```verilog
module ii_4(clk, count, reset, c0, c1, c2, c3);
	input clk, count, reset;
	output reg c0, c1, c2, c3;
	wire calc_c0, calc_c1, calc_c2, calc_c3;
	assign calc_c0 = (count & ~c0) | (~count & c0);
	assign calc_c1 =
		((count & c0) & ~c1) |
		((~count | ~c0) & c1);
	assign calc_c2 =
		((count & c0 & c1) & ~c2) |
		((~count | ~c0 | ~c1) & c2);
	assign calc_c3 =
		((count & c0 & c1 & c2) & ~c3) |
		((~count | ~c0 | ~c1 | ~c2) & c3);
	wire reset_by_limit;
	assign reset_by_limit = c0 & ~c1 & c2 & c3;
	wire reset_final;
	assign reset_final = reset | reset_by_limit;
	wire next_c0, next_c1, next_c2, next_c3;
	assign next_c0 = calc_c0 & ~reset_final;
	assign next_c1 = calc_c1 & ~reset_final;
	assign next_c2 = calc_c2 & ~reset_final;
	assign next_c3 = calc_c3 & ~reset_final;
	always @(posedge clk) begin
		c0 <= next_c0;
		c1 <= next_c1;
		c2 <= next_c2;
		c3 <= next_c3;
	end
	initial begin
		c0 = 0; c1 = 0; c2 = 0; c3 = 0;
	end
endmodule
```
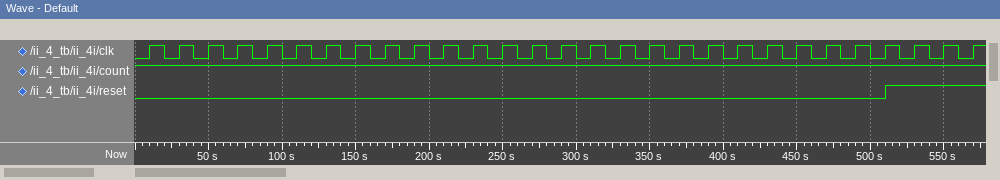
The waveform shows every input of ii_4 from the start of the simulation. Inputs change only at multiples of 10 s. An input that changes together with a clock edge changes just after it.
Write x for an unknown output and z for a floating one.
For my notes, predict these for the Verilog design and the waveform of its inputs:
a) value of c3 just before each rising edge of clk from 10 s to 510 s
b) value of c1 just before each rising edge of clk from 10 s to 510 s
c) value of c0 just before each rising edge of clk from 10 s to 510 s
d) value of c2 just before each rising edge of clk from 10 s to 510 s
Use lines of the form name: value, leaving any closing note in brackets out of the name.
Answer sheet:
value of c3 just before each rising edge of clk from 10 s to 510 s: 0 0 0 0 0 0 0 0 1 1 1 1 1 1 0 0 0 0 0 0 0 0 1 1 1 1
value of c1 just before each rising edge of clk from 10 s to 510 s: 0 0 1 1 0 0 1 1 0 0 1 1 0 0 0 0 1 1 0 0 1 1 0 0 1 1
value of c0 just before each rising edge of clk from 10 s to 510 s: 0 1 0 1 0 1 0 1 0 1 0 1 0 1 0 1 0 1 0 1 0 1 0 1 0 1
value of c2 just before each rising edge of clk from 10 s to 510 s: 0 0 0 0 1 1 1 1 0 0 0 0 1 1 0 0 0 0 1 1 1 1 0 0 0 0
